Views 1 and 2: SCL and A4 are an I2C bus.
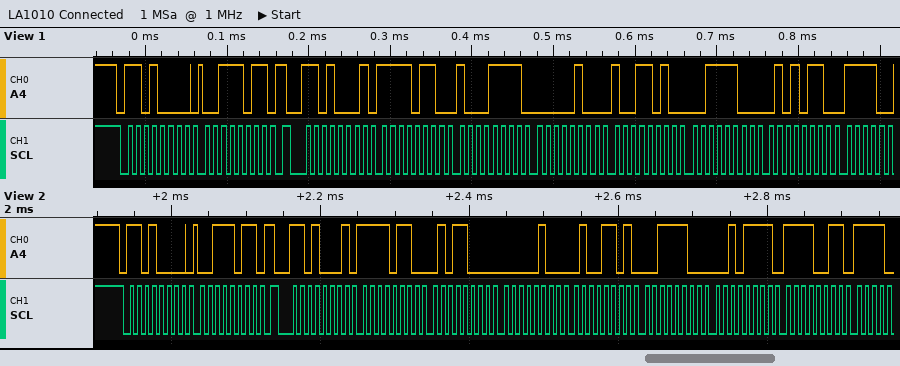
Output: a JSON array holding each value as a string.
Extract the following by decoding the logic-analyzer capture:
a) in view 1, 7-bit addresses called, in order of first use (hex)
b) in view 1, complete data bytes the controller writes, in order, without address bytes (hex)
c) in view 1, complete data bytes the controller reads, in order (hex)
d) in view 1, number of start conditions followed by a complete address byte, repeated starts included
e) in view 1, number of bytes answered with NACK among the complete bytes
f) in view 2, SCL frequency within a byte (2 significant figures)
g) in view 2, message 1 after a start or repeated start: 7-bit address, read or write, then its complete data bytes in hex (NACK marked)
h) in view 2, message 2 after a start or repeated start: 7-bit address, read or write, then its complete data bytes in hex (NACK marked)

["0x68", "3B", "F6 8F 04 9A 3C 56", "2", "0", "100 kHz", "0x68 write: 3B", "0x68 read: F6 58 04 4D 3C 2F F3"]
